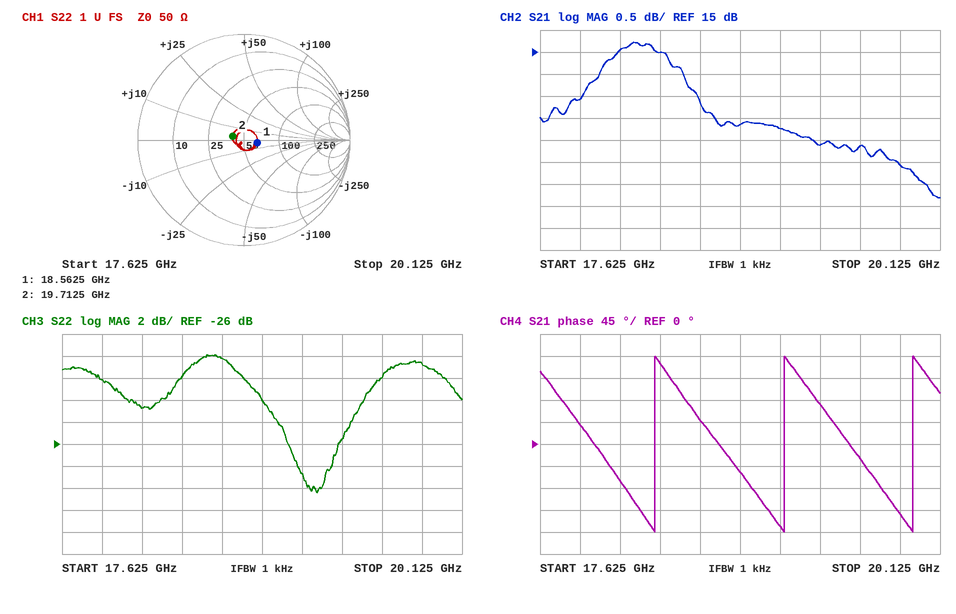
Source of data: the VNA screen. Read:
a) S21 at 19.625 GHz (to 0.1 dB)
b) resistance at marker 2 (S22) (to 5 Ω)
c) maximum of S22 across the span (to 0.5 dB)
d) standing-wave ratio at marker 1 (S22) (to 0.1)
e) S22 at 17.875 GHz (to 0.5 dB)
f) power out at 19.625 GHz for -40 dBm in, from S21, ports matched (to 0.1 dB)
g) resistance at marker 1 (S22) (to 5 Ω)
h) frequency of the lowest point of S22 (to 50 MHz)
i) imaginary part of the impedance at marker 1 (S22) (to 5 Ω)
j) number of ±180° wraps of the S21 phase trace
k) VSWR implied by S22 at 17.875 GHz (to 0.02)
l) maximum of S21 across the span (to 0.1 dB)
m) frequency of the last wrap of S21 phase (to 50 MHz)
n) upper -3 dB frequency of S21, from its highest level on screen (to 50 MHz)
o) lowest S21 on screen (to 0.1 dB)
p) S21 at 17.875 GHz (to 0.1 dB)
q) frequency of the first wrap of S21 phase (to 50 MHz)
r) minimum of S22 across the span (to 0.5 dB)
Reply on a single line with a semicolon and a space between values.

12.9 dB; 40 Ω; -18.0 dB; 1.3; -20.0 dB; -27.1 dBm; 65 Ω; 19.20 GHz; -5 Ω; 3; 1.22; 15.2 dB; 19.95 GHz; 19.95 GHz; 11.7 dB; 13.9 dB; 18.35 GHz; -30.5 dB
